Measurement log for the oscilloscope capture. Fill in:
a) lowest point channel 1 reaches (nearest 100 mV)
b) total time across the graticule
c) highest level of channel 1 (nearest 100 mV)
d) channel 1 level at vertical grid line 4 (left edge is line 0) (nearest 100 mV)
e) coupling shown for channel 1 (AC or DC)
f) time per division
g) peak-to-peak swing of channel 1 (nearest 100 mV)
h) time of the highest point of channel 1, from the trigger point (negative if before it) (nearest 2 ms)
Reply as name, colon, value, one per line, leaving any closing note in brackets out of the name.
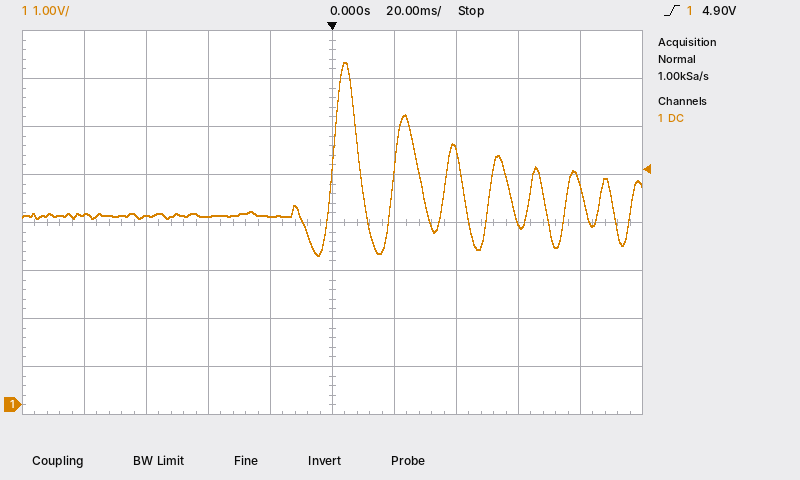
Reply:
lowest point channel 1 reaches: 3.1 V
total time across the graticule: 200 ms
highest level of channel 1: 7.1 V
channel 1 level at vertical grid line 4 (left edge is line 0): 3.9 V
coupling shown for channel 1: DC
time per division: 20 ms
peak-to-peak swing of channel 1: 4.0 V
time of the highest point of channel 1, from the trigger point (negative if before it): +4 ms
